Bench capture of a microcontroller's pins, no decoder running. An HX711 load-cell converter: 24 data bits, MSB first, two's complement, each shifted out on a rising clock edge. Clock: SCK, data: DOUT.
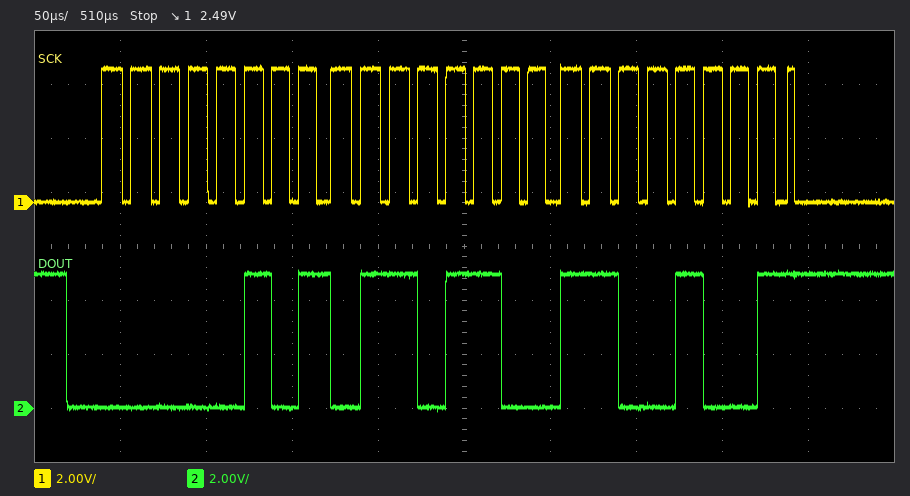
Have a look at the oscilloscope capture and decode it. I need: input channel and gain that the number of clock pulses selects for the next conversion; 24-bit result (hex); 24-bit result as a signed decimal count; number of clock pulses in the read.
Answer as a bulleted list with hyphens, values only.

- channel A, gain 128
- 0x056CC9
- 355529
- 25
